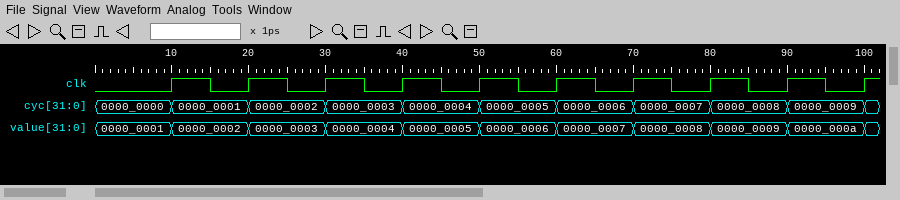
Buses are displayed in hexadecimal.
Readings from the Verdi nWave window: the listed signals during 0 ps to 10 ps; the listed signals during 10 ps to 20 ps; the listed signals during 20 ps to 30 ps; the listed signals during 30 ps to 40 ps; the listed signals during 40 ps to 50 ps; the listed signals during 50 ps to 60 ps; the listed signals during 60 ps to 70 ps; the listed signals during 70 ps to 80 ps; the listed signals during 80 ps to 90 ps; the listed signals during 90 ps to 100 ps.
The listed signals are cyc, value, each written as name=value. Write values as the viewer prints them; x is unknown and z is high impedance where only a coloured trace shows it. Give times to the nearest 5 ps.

cyc=0000_0000, value=0000_0001
cyc=0000_0001, value=0000_0002
cyc=0000_0002, value=0000_0003
cyc=0000_0003, value=0000_0004
cyc=0000_0004, value=0000_0005
cyc=0000_0005, value=0000_0006
cyc=0000_0006, value=0000_0007
cyc=0000_0007, value=0000_0008
cyc=0000_0008, value=0000_0009
cyc=0000_0009, value=0000_000a
